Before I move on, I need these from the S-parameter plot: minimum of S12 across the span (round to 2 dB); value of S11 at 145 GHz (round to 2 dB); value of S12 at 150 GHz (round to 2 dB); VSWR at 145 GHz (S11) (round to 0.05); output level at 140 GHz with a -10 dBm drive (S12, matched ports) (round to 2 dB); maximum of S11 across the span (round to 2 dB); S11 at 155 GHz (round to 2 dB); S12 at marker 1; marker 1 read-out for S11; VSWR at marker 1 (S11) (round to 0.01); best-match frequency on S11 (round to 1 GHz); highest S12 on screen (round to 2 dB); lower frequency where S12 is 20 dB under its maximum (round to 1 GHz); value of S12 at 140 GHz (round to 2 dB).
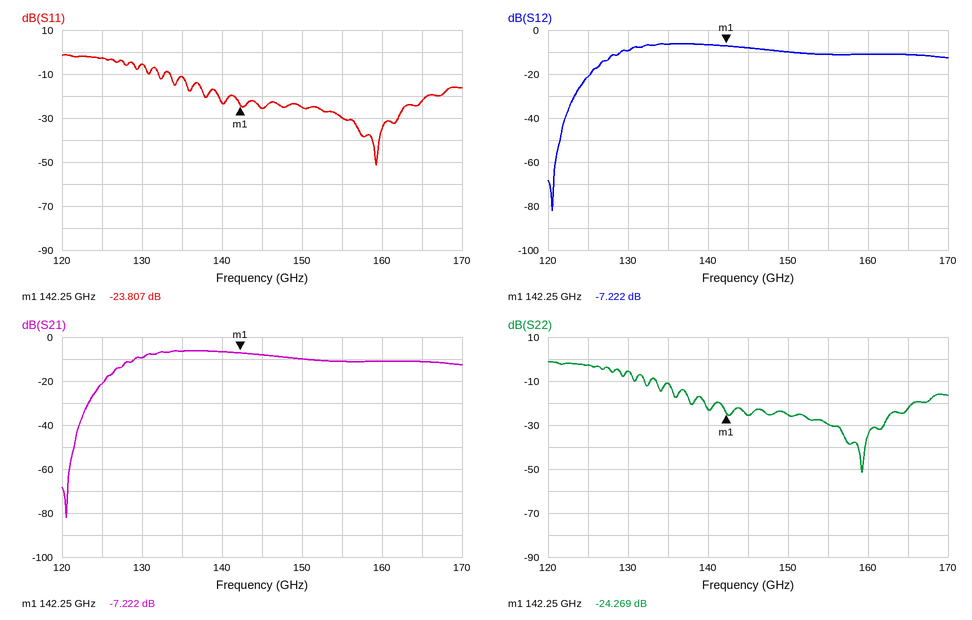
-82 dB
-26 dB
-10 dB
1.10
-16 dBm
-2 dB
-30 dB
-7.222 dB
-23.807 dB
1.14
159 GHz
-6 dB
124 GHz
-6 dB
